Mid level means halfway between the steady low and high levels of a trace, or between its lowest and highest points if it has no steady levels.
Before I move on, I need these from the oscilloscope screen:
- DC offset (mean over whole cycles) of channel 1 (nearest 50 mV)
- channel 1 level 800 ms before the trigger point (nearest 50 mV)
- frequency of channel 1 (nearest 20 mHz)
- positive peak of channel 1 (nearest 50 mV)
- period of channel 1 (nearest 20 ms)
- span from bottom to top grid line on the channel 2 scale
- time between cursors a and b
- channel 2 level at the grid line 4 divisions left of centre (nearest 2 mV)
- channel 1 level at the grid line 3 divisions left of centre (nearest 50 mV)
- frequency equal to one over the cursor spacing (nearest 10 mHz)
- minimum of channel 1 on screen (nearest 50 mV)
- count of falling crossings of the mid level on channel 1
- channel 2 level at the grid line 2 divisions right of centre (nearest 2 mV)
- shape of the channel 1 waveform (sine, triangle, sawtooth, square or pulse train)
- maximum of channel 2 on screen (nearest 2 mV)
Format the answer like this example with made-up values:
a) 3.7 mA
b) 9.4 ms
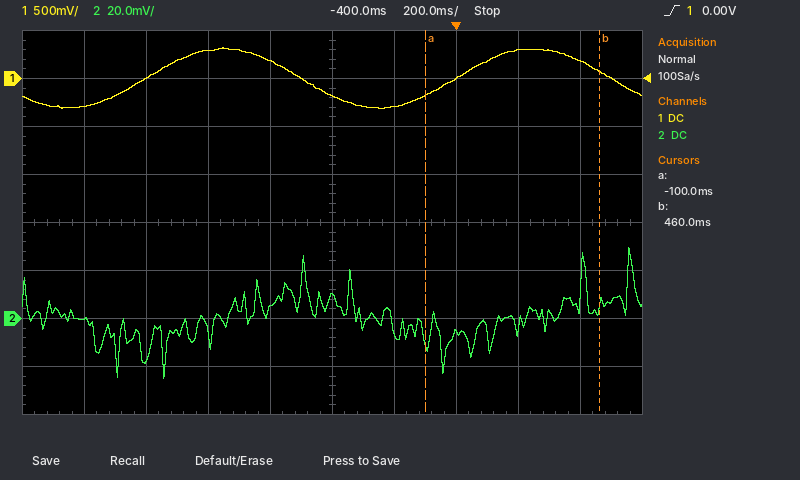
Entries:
a) 0 mV
b) 300 mV
c) 1.00 Hz
d) 300 mV
e) 1.00 s
f) 160 mV
g) 560 ms
h) 0 mV
i) 0 mV
j) 1.79 Hz
k) -300 mV
l) 2
m) -6 mV
n) sine
o) 30 mV
